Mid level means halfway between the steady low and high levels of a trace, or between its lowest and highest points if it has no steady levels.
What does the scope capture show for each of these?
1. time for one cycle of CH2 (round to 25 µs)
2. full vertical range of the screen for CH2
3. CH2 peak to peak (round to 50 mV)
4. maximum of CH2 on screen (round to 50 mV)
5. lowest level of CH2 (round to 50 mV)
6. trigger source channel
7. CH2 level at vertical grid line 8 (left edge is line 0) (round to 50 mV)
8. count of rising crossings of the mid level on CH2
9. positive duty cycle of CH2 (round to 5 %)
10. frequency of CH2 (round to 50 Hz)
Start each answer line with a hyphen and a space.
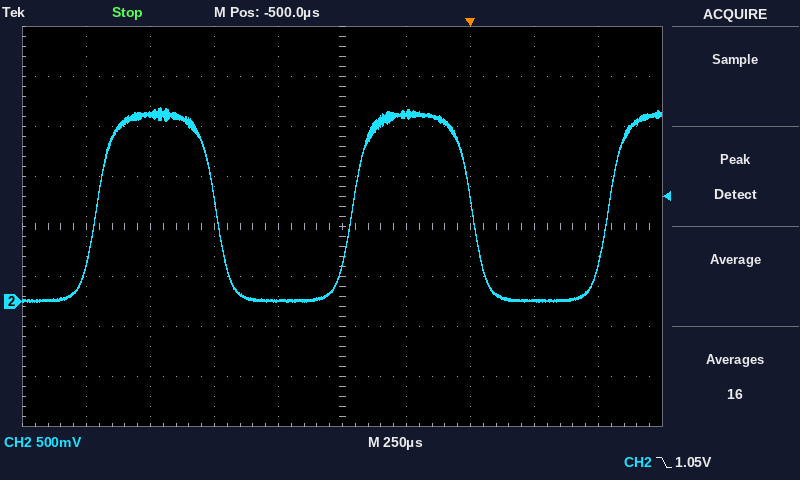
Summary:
- 1.000 ms
- 4 V
- 1.95 V
- 1.95 V
- 0 mV
- CH2
- 0 mV
- 3
- 45 %
- 1.00 kHz
